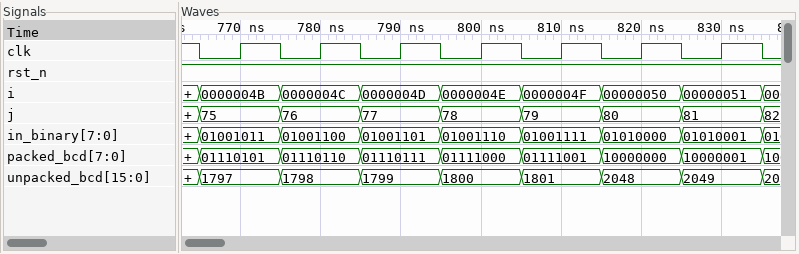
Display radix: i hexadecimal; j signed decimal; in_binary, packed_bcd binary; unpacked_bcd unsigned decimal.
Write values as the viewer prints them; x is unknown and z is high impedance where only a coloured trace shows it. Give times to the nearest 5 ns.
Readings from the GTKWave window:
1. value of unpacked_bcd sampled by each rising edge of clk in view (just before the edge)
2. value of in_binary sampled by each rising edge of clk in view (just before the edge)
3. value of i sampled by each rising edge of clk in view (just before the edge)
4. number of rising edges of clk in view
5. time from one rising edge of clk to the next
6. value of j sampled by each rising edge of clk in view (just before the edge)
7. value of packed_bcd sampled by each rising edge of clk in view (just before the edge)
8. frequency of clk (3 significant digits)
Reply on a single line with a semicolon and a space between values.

1797, 1798, 1799, 1800, 1801, 2048, 2049; 01001011, 01001100, 01001101, 01001110, 01001111, 01010000, 01010001; 0000004B, 0000004C, 0000004D, 0000004E, 0000004F, 00000050, 00000051; 7; 10 ns; 75, 76, 77, 78, 79, 80, 81; 01110101, 01110110, 01110111, 01111000, 01111001, 10000000, 10000001; 100 MHz
